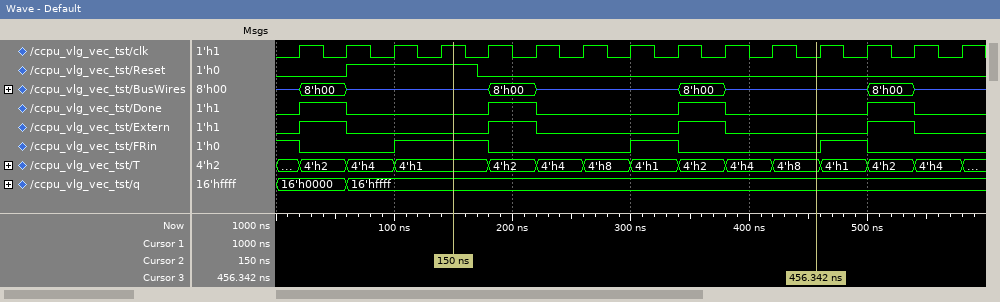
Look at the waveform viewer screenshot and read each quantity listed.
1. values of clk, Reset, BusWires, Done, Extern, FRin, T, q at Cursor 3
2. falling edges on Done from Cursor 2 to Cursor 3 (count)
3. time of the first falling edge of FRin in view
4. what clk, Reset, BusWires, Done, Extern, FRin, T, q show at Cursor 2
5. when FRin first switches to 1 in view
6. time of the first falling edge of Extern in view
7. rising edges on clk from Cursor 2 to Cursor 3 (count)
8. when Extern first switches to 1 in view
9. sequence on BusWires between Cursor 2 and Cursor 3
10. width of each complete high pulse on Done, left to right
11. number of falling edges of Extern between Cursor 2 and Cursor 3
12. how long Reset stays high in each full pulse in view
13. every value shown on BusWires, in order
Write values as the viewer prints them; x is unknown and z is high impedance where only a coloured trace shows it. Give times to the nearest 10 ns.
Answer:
clk=0, Reset=0, BusWires=z, Done=0, Extern=0, FRin=0, T=4'h8, q=16'hffff
2
20 ns
clk=1, Reset=1, BusWires=z, Done=0, Extern=0, FRin=1, T=4'h1, q=16'hffff
100 ns
60 ns
7
20 ns
z, 8'h00, z, 8'h00, z
40 ns, 40 ns, 40 ns, 40 ns
2
110 ns
z, 8'h00, z, 8'h00, z, 8'h00, z, 8'h00, z
